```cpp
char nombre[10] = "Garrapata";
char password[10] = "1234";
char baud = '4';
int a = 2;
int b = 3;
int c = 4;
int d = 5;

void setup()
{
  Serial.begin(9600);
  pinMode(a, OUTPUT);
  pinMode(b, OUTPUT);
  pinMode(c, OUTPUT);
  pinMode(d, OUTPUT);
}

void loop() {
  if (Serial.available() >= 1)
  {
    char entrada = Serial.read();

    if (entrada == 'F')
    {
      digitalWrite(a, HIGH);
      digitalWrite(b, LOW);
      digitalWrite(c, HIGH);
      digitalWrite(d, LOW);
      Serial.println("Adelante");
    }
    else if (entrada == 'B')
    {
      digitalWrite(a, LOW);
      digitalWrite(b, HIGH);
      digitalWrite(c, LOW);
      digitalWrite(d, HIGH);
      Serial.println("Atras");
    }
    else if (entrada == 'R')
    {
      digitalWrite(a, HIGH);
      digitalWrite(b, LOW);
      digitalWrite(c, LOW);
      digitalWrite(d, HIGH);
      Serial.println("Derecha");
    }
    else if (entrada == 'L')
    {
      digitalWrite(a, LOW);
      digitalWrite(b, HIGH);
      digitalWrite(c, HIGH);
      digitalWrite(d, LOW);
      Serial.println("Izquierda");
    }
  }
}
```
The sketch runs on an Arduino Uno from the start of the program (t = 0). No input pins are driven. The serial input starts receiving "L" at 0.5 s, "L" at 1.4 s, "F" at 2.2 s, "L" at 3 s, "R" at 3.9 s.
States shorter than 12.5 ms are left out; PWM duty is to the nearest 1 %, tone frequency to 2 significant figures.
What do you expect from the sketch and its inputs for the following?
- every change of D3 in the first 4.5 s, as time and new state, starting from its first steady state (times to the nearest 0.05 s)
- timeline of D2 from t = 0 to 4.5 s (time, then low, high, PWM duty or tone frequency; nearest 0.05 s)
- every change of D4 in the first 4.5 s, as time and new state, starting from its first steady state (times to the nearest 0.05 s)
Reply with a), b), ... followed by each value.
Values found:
a) 0 s low; 0.5 s high; 2.2 s low; 3 s high; 3.9 s low
b) 0 s low; 2.2 s high; 3 s low; 3.9 s high
c) 0 s low; 0.5 s high; 3.9 s low
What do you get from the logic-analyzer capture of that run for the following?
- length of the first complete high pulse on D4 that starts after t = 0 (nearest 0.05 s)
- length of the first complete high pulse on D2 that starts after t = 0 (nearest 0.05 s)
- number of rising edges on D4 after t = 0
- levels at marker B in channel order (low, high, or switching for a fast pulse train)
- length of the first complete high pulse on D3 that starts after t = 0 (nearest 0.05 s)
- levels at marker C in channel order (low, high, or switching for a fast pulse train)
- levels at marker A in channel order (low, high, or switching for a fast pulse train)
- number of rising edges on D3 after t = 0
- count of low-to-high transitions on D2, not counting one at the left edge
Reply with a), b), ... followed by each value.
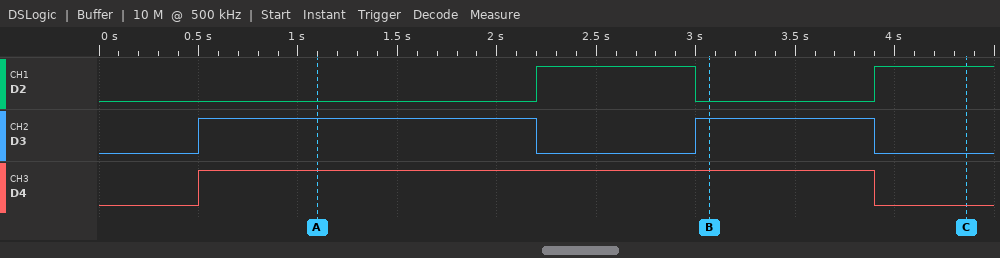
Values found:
a) 3.40 s
b) 0.80 s
c) 1
d) D2 low, D3 high, D4 high
e) 1.70 s
f) D2 high, D3 low, D4 low
g) D2 low, D3 high, D4 high
h) 2
i) 2
